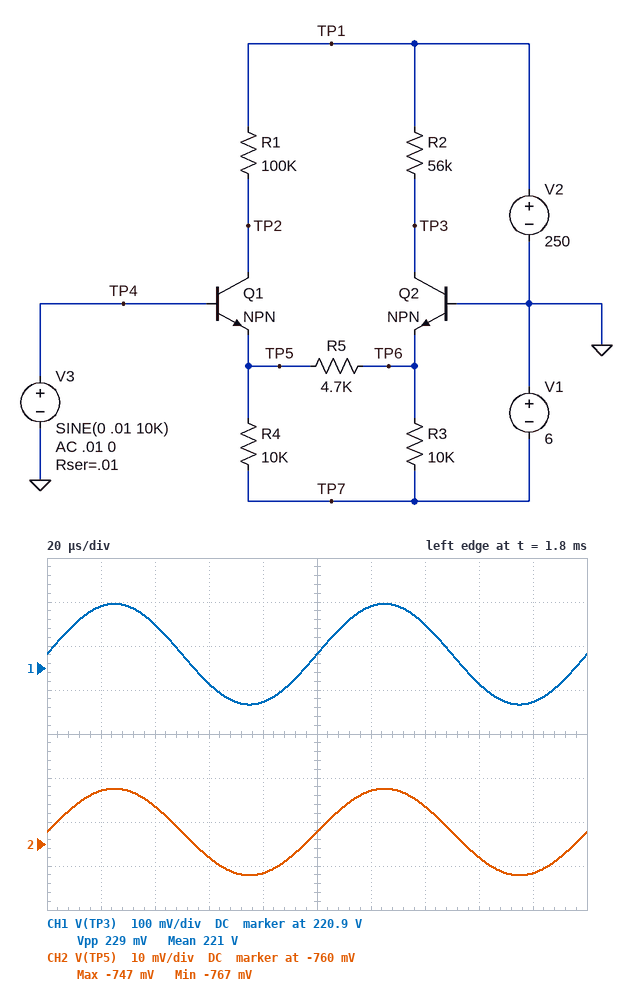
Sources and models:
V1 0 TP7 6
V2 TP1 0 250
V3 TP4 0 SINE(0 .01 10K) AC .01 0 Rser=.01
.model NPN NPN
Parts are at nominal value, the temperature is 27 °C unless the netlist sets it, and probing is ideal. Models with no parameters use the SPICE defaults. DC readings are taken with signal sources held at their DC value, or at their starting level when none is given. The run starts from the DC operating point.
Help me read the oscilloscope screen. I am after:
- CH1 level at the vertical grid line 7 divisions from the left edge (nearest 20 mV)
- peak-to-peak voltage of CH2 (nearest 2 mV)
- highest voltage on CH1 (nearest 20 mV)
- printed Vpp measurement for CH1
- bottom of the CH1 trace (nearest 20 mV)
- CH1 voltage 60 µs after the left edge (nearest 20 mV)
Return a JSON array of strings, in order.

["221.00 V", "20 mV", "221.04 V", "229 mV", "220.82 V", "220.86 V"]
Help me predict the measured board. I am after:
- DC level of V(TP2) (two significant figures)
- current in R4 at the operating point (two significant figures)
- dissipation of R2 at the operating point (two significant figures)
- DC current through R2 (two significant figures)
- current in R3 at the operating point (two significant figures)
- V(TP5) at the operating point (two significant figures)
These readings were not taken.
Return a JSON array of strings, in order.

["200 V", "520 µA", "15 mW", "520 µA", "520 µA", "-760 mV"]
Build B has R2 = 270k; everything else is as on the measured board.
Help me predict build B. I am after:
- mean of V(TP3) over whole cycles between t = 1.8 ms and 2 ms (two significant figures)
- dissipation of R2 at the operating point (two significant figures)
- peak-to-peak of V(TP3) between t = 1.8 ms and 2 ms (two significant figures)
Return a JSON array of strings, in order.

["110 V", "73 mW", "1.1 V"]
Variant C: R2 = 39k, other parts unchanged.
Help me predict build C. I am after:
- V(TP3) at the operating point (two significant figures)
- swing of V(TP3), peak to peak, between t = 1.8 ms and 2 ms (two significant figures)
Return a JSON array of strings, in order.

["230 V", "160 mV"]
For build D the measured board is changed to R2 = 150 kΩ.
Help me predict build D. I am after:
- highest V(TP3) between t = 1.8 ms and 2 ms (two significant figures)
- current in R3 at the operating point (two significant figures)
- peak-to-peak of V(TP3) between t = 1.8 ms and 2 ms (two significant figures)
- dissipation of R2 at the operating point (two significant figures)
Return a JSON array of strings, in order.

["170 V", "520 µA", "610 mV", "40 mW"]
